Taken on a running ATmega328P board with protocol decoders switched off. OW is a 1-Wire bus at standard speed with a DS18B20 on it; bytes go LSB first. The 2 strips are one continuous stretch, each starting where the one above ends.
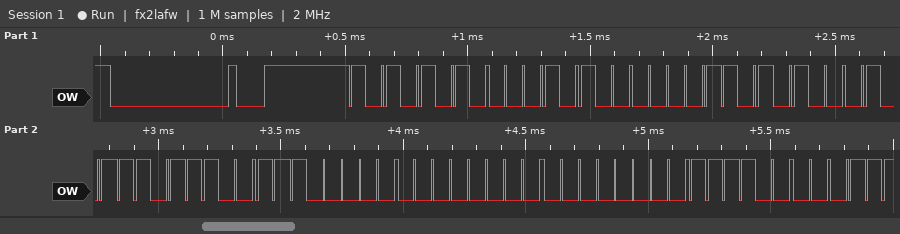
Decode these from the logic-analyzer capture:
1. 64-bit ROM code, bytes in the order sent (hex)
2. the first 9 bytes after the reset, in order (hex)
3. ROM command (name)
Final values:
28 B0 A2 3B 07 00 00 0F
55 28 B0 A2 3B 07 00 00 0F
Match ROM
